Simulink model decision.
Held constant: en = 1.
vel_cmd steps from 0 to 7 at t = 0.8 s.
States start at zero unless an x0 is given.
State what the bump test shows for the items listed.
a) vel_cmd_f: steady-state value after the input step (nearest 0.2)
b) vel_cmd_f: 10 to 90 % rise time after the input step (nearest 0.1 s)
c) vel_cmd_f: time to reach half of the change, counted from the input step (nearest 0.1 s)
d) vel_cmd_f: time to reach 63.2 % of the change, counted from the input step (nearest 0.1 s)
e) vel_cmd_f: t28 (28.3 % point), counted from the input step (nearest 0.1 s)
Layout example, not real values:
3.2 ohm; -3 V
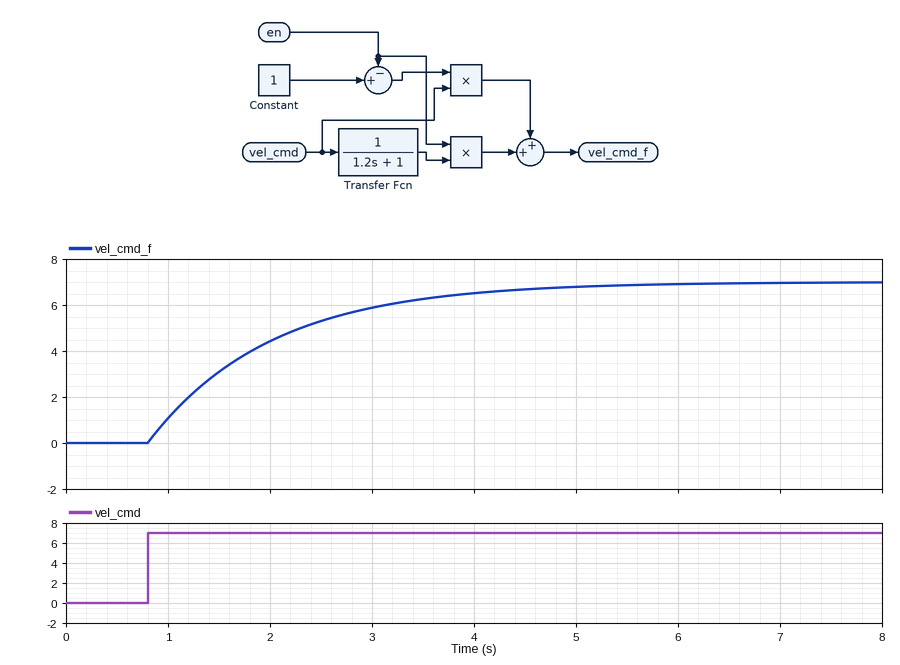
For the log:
7.0; 2.6 s; 0.8 s; 1.2 s; 0.4 s
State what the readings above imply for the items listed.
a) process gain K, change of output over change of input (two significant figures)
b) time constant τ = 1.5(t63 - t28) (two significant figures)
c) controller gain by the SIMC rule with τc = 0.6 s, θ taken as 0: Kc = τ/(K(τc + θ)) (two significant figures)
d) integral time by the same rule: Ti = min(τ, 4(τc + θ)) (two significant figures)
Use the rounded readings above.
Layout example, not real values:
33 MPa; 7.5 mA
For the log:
1.0; 1.2 s; 2.0; 1.2 s
